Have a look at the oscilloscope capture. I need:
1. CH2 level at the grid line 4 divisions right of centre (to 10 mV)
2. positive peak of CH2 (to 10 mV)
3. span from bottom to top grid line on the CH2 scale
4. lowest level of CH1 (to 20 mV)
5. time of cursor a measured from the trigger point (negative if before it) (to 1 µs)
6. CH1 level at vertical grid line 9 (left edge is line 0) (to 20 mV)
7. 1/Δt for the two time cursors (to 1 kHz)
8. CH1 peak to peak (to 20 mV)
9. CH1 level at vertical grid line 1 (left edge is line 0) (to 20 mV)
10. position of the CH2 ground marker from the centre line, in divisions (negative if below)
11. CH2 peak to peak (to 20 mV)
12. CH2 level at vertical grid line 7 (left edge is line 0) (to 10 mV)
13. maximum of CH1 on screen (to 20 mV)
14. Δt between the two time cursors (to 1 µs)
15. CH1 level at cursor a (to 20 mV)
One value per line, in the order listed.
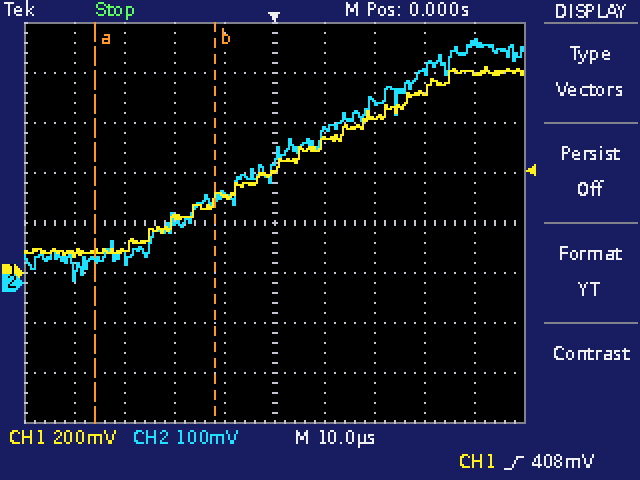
480 mV
490 mV
800 mV
60 mV
-36 µs
800 mV
42 kHz
760 mV
80 mV
-1.2 div
480 mV
360 mV
820 mV
24 µs
80 mV
